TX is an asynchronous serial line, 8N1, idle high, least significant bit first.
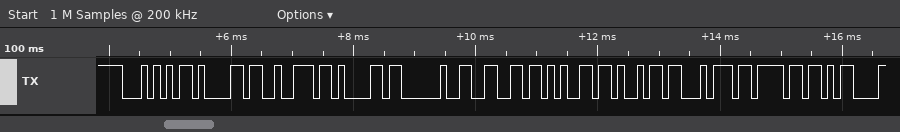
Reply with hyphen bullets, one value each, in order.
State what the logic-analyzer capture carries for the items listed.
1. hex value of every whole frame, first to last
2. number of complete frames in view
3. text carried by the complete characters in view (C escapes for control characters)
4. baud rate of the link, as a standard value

- 0x54 0x61 0x72 0x61 0x20 0x66 0x65 0x69 0x74 0x6F 0x0D
- 11
- "Tara feito\r"
- 9600 baud
